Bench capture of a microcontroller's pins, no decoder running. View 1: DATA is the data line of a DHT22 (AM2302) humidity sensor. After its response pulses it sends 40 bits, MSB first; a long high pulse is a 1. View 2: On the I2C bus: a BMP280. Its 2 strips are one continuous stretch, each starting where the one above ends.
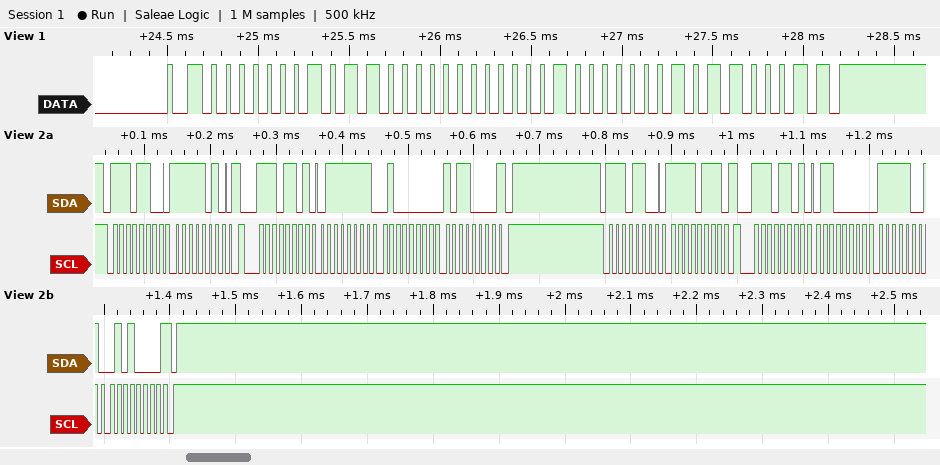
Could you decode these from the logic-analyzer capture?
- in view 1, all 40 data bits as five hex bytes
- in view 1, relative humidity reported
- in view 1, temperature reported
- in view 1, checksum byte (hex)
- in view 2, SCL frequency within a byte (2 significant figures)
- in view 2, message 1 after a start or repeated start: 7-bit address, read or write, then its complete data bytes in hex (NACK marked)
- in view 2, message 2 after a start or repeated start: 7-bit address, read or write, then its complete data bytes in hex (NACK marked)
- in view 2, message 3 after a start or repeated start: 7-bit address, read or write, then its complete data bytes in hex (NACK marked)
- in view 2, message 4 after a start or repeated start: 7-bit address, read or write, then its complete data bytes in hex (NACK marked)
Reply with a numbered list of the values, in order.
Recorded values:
1. 01 60 01 01 63
2. 35.2 %
3. 25.7 °C
4. 0x63
5. 100 kHz
6. 0x76 write: FA
7. 0x76 read: 7F 40 B0 NACK
8. 0x76 write: F7
9. 0x76 read: 60 F9 50 NACK
